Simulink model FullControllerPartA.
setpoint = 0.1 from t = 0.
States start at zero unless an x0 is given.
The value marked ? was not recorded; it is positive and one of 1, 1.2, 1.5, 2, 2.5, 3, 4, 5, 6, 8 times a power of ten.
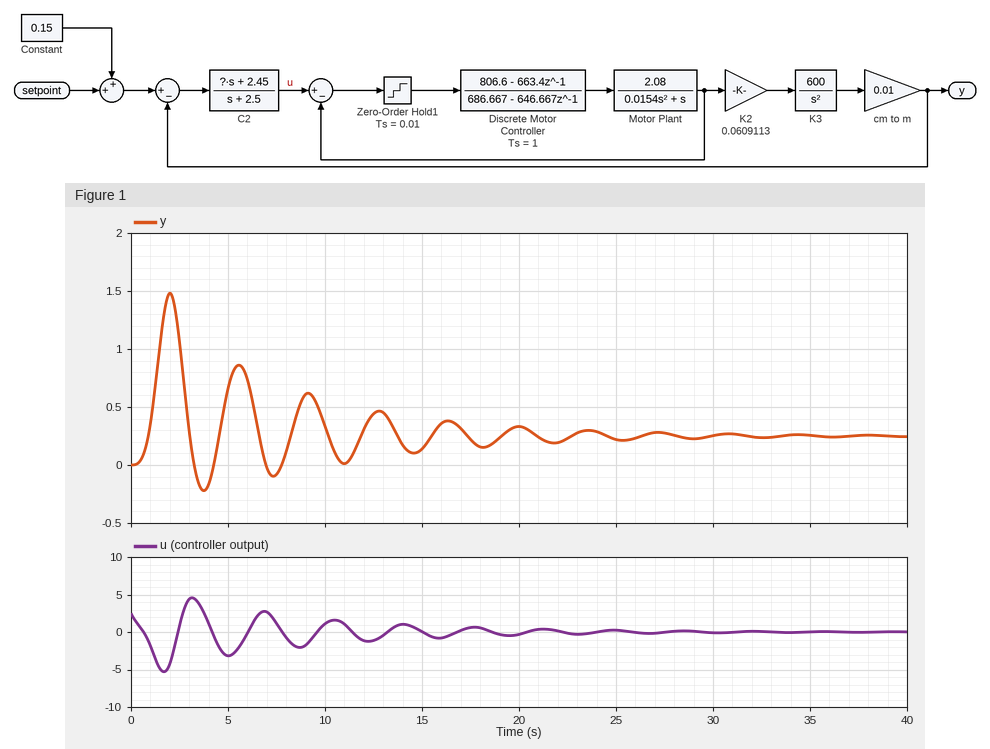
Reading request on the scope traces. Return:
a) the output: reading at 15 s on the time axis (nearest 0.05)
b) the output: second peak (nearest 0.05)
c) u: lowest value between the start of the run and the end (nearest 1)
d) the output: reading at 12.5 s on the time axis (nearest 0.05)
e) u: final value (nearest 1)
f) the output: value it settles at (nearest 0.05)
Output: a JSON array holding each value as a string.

["0.15", "0.85", "-5", "0.45", "0", "0.25"]
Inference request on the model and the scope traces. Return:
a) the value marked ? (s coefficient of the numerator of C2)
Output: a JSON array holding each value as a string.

["10"]
